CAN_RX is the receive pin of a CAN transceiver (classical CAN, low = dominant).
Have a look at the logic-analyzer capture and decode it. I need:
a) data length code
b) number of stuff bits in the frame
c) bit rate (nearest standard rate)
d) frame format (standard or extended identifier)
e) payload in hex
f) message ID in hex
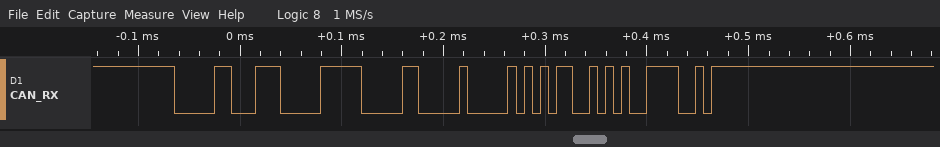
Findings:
3
6
125 kbit/s
standard
C2 00 2B
0x047
